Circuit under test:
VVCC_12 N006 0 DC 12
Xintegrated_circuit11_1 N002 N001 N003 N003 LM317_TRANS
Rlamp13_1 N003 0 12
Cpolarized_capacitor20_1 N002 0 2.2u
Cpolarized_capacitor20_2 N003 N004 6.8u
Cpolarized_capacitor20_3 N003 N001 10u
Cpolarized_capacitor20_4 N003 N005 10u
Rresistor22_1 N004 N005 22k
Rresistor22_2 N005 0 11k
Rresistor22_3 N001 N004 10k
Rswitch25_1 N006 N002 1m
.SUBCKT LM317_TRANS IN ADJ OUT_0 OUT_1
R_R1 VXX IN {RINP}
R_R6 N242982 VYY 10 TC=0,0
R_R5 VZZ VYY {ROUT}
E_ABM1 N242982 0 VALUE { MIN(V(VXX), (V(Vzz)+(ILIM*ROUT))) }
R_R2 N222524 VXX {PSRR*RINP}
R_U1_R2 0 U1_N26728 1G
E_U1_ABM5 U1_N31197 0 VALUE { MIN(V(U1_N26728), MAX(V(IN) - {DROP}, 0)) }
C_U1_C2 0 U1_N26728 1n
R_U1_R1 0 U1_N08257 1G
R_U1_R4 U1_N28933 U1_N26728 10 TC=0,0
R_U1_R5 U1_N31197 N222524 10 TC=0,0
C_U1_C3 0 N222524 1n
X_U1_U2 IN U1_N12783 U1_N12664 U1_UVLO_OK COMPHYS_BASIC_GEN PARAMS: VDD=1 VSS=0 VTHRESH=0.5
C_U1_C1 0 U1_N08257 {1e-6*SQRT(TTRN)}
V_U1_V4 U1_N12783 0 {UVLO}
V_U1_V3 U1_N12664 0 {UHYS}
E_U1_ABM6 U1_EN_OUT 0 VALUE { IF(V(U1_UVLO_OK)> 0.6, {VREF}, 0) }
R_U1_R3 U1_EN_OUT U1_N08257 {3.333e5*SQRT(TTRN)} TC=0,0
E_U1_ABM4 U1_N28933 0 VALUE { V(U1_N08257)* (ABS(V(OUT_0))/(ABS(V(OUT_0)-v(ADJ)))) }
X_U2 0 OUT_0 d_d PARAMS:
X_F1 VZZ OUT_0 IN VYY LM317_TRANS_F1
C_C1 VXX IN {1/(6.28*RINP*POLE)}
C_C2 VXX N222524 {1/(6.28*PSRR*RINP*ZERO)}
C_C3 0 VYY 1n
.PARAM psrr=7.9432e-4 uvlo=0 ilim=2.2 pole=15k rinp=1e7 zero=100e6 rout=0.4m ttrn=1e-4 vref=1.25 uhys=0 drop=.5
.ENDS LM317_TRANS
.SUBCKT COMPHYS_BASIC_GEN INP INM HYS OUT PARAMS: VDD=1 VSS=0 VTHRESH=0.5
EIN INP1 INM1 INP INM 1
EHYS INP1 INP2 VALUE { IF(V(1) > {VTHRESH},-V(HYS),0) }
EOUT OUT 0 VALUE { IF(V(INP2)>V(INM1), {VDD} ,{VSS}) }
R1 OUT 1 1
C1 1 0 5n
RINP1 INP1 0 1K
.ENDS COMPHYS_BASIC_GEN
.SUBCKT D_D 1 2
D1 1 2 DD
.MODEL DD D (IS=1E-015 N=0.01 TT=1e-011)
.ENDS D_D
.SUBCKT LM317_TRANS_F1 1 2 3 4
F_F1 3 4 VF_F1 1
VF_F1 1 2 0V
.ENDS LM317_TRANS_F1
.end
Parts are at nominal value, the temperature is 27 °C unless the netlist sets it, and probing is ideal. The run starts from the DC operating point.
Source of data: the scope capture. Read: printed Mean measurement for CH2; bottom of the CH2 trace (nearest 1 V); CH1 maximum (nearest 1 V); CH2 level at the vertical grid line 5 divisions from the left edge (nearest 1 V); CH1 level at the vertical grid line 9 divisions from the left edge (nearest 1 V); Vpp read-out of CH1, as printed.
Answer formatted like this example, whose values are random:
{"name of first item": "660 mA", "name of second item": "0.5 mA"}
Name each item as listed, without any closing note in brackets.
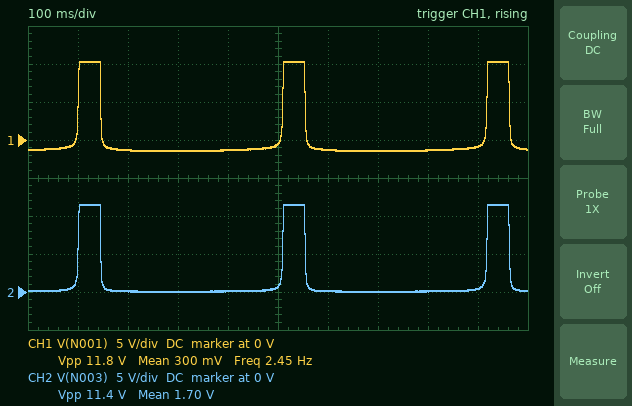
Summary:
{"printed Mean measurement for CH2": "1.70 V", "bottom of the CH2 trace": "0 V", "CH1 maximum": "10 V", "CH2 level at the vertical grid line 5 divisions from the left edge": "1 V", "CH1 level at the vertical grid line 9 divisions from the left edge": "-1 V", "Vpp read-out of CH1, as printed": "11.8 V"}
